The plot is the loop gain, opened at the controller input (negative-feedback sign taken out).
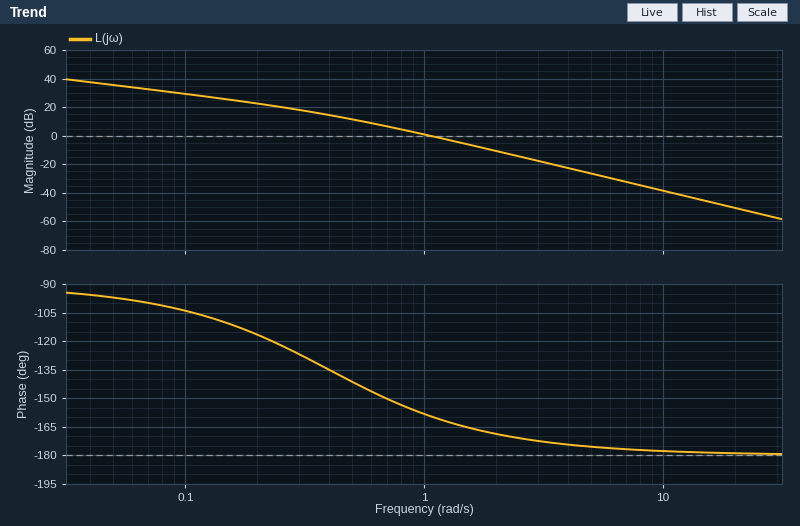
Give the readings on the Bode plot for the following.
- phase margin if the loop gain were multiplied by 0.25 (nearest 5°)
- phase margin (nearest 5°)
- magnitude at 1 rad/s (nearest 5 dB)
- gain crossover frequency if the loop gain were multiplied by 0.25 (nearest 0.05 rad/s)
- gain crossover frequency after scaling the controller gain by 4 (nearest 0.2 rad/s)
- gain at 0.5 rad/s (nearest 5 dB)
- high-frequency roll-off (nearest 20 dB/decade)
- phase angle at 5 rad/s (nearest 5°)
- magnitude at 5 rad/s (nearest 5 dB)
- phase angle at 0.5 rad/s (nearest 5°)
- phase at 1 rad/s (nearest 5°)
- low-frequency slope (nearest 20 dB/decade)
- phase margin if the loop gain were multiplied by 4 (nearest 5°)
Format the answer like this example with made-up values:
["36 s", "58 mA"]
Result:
["40°", "20°", "0 dB", "0.50 rad/s", "2.2 rad/s", "10 dB", "-40 dB/decade", "-175°", "-25 dB", "-140°", "-160°", "-20 dB/decade", "10°"]
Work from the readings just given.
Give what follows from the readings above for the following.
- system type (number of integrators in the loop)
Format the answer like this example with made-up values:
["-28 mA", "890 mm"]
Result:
["1"]
